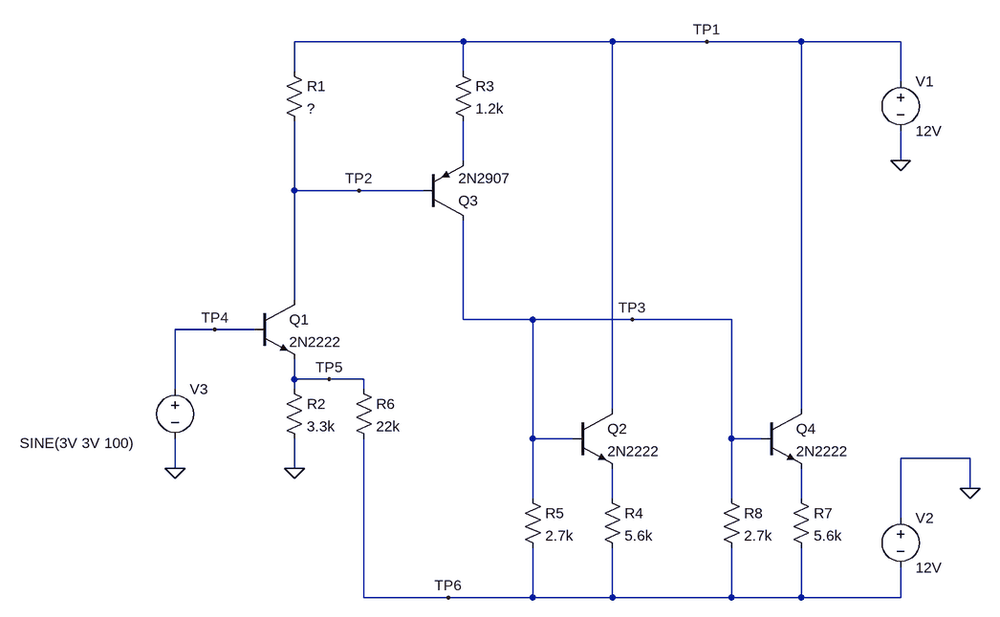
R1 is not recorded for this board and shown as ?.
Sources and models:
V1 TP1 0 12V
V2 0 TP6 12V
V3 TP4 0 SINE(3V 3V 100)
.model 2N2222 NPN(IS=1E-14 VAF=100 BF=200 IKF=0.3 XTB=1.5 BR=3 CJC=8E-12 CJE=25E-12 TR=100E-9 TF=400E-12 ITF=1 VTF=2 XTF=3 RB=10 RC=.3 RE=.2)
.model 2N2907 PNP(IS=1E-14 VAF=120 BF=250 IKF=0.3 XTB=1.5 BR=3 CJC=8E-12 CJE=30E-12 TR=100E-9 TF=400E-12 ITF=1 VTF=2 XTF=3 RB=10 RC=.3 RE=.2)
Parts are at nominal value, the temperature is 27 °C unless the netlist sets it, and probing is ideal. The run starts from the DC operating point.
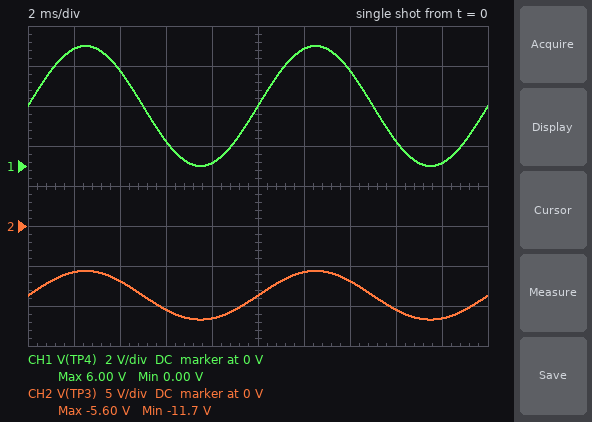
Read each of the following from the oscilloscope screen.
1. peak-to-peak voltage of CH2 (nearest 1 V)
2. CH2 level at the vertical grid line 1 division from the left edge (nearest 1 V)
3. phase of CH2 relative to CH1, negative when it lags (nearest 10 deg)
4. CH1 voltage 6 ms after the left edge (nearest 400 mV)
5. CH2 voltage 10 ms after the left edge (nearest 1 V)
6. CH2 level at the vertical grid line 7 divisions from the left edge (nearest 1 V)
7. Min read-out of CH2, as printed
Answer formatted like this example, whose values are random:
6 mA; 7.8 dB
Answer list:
6 V; -6 V; 0 deg; 1.2 V; -9 V; -7 V; -11.7 V
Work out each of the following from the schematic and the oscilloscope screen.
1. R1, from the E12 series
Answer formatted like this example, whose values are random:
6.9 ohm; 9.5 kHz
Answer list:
2.7 kΩ
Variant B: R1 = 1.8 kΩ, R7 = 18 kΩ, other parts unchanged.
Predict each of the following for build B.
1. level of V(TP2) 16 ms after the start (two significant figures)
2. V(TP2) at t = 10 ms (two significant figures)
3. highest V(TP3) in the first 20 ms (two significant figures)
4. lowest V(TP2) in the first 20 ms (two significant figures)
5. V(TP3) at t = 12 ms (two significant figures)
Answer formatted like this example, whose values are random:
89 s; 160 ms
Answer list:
11 V; 9.6 V; -8.0 V; 7.7 V; -8.1 V
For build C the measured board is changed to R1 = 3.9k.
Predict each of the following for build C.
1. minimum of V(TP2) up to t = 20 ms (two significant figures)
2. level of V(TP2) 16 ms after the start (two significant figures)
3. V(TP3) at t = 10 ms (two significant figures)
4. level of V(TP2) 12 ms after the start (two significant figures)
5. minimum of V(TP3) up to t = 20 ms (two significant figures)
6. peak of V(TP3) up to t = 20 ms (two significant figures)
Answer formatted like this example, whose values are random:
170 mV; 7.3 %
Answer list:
4.3 V; 9.1 V; -6.9 V; 5.2 V; -11 V; -4.2 V
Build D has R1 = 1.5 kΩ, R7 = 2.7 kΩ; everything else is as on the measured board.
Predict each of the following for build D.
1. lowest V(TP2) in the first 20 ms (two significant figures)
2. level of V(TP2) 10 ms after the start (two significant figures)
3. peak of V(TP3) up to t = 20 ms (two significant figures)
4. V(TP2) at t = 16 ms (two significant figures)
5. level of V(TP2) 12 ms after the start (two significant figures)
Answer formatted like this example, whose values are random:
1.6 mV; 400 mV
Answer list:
8.4 V; 10 V; -8.8 V; 11 V; 8.5 V
